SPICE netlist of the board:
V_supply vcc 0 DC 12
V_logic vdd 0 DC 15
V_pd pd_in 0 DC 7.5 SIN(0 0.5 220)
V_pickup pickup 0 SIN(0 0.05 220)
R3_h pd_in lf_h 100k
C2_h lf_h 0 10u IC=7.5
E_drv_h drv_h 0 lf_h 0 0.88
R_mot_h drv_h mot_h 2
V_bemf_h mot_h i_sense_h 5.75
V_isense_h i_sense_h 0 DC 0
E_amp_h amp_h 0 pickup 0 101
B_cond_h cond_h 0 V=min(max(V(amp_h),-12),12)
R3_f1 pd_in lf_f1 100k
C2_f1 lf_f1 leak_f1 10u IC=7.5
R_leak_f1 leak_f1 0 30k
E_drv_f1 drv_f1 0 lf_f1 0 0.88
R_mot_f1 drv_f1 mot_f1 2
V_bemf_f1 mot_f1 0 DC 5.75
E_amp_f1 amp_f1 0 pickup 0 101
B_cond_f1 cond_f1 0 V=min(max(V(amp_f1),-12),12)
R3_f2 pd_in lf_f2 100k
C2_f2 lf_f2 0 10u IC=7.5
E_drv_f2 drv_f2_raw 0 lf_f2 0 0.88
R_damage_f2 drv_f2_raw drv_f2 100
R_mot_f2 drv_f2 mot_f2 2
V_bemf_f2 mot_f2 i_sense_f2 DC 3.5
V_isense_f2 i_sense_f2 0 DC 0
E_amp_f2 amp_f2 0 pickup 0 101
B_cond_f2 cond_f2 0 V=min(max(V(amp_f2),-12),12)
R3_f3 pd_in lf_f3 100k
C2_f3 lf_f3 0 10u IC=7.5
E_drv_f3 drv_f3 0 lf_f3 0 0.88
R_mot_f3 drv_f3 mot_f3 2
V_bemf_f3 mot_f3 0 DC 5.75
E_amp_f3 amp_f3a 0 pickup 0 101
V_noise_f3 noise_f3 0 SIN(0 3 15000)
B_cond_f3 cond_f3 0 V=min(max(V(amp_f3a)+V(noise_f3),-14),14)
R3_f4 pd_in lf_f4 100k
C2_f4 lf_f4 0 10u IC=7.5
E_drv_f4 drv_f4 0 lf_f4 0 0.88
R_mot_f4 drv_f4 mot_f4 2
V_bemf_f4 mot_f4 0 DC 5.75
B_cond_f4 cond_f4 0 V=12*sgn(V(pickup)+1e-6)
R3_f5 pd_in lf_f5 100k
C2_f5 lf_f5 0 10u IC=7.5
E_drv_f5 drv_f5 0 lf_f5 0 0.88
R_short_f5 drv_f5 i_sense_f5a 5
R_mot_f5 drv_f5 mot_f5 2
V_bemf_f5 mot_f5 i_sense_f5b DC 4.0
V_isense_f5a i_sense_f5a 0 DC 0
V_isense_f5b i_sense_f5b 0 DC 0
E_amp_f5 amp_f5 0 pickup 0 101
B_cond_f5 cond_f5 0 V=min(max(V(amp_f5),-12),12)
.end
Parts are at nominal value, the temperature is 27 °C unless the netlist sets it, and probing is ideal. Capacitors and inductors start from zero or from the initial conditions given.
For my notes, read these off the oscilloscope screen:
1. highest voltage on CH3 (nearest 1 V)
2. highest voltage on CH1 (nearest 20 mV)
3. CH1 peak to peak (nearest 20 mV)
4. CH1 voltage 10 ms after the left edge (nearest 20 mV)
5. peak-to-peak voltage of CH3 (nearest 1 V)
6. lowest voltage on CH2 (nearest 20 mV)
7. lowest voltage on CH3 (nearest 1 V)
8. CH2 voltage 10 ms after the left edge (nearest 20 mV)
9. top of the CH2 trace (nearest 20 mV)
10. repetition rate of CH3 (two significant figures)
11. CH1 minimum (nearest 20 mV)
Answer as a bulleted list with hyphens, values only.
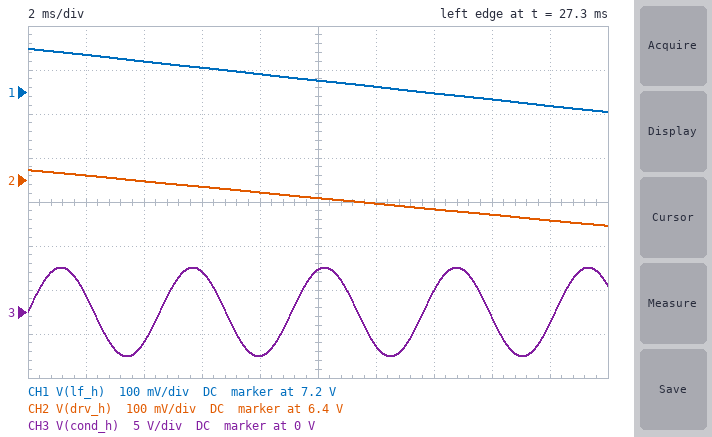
- 5 V
- 7.30 V
- 140 mV
- 7.22 V
- 10 V
- 6.30 V
- -5 V
- 6.36 V
- 6.42 V
- 220 Hz
- 7.16 V
